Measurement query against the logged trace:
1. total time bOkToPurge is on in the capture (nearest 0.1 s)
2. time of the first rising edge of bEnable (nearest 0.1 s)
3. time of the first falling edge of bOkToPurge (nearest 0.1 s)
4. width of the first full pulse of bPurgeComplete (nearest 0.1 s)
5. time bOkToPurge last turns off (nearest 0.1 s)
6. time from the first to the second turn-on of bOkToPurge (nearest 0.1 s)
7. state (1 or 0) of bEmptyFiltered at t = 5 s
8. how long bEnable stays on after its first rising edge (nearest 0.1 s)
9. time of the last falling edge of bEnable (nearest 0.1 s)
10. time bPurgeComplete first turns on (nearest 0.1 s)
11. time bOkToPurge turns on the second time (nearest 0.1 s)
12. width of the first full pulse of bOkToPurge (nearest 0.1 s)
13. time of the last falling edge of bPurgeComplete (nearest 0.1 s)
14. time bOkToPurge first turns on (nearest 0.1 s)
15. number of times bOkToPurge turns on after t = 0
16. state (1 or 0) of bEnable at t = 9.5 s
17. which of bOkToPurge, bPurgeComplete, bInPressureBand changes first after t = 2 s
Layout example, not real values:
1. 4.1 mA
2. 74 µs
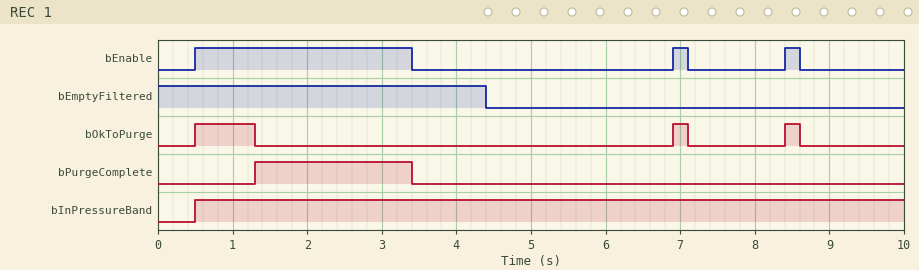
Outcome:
1. 1.2 s
2. 0.5 s
3. 1.3 s
4. 2.1 s
5. 8.6 s
6. 6.4 s
7. 0
8. 2.9 s
9. 8.6 s
10. 1.3 s
11. 6.9 s
12. 0.8 s
13. 3.4 s
14. 0.5 s
15. 3
16. 0
17. bPurgeComplete
